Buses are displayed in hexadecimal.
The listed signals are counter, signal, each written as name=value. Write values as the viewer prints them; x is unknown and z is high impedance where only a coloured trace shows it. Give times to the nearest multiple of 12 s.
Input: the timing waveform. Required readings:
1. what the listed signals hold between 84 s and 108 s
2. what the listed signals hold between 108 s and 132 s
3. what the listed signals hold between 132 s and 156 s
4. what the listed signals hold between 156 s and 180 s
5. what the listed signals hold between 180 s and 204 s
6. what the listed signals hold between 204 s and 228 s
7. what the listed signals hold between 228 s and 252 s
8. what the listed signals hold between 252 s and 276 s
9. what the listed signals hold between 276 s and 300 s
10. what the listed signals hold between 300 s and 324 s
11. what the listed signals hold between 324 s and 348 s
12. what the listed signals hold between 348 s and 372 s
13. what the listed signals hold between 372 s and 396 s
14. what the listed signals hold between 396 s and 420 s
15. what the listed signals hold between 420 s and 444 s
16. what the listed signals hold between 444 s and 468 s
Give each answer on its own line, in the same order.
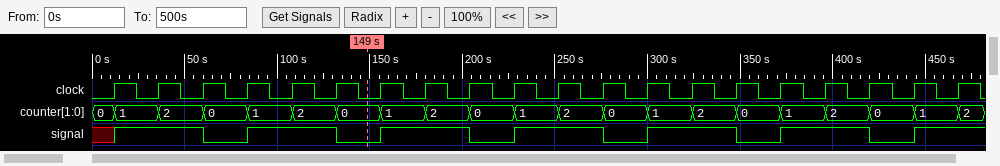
counter=1, signal=1
counter=2, signal=1
counter=0, signal=0
counter=1, signal=1
counter=2, signal=1
counter=0, signal=0
counter=1, signal=1
counter=2, signal=1
counter=0, signal=0
counter=1, signal=1
counter=2, signal=1
counter=0, signal=0
counter=1, signal=1
counter=2, signal=1
counter=0, signal=0
counter=1, signal=1
